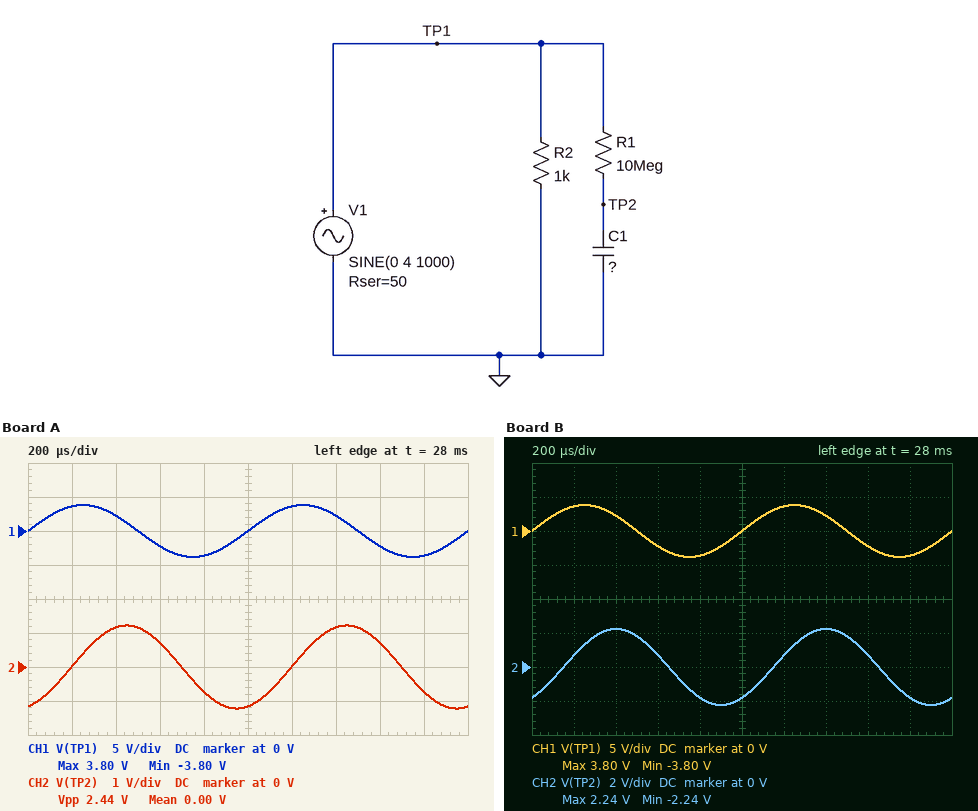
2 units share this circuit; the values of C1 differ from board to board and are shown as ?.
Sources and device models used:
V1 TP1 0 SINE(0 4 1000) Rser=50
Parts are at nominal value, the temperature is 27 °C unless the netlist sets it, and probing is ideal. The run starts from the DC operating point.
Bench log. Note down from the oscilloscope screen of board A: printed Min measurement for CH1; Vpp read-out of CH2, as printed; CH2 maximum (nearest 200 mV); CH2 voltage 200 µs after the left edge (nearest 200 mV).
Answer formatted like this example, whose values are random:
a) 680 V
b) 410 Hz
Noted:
a) -3.80 V
b) 2.44 V
c) 1.2 V
d) 0 V
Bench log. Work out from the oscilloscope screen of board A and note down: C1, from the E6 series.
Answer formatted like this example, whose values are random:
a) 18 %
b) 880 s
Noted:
a) 47 pF
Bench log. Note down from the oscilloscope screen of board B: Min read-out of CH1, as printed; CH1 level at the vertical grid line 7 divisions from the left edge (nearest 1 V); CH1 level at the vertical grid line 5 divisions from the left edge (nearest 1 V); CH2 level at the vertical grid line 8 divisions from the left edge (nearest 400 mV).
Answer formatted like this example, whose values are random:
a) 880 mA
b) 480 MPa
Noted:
a) -3.80 V
b) 2 V
c) 0 V
d) 800 mV
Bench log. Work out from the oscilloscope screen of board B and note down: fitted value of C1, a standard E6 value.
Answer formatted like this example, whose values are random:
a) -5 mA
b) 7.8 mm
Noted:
a) 22 pF
